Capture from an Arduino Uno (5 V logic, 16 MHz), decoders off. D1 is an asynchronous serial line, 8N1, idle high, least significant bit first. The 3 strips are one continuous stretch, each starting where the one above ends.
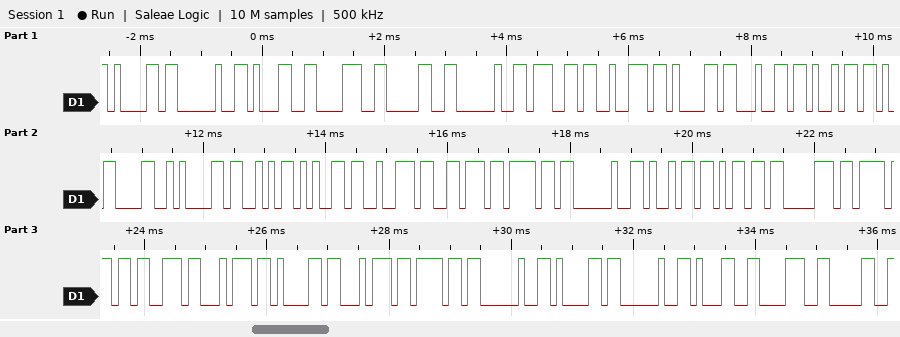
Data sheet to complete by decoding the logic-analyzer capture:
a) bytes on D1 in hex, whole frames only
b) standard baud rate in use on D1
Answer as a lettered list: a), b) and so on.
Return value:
a) 61 20 31 38 30 20 67 72 61 64 69 0D 0A 53 65 72 76 6F 20 69 6D 70 6F 73 74 61 74 6F 20 61 20 31 38 30
b) 9600 baud
